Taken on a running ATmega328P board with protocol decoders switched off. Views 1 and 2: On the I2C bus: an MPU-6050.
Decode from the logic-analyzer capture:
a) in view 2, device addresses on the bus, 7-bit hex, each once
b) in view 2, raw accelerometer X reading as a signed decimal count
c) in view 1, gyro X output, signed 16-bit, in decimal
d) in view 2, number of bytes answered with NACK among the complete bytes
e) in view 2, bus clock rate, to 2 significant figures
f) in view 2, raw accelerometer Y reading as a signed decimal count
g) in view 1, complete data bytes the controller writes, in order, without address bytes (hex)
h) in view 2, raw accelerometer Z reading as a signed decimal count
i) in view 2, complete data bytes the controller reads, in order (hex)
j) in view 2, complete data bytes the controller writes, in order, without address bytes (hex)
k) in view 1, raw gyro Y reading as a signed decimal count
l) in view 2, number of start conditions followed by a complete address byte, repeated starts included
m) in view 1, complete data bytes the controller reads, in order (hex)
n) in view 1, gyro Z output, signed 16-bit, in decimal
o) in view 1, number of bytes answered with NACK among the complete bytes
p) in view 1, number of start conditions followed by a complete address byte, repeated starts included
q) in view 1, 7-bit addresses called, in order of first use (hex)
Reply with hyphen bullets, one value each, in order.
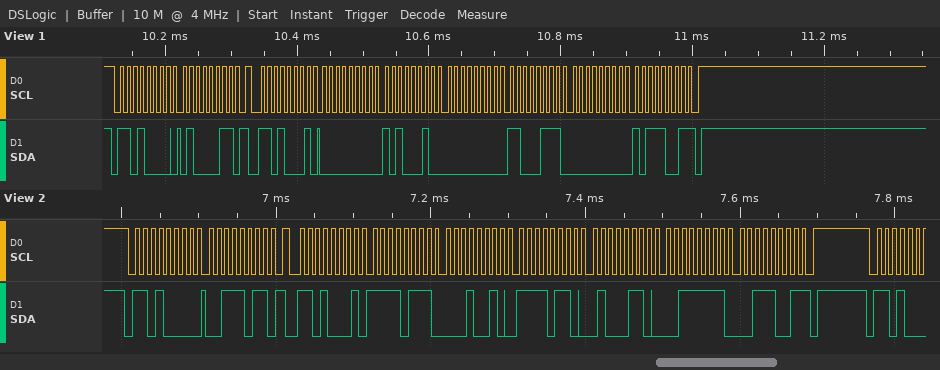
- 0x68
- -2286
- 162
- 1
- 100 kHz
- -2490
- 43
- 16185
- F7 12 F6 46 3F 39
- 3B
- 199
- 2
- 00 A2 00 C7 00 B9
- 185
- 1
- 2
- 0x68
